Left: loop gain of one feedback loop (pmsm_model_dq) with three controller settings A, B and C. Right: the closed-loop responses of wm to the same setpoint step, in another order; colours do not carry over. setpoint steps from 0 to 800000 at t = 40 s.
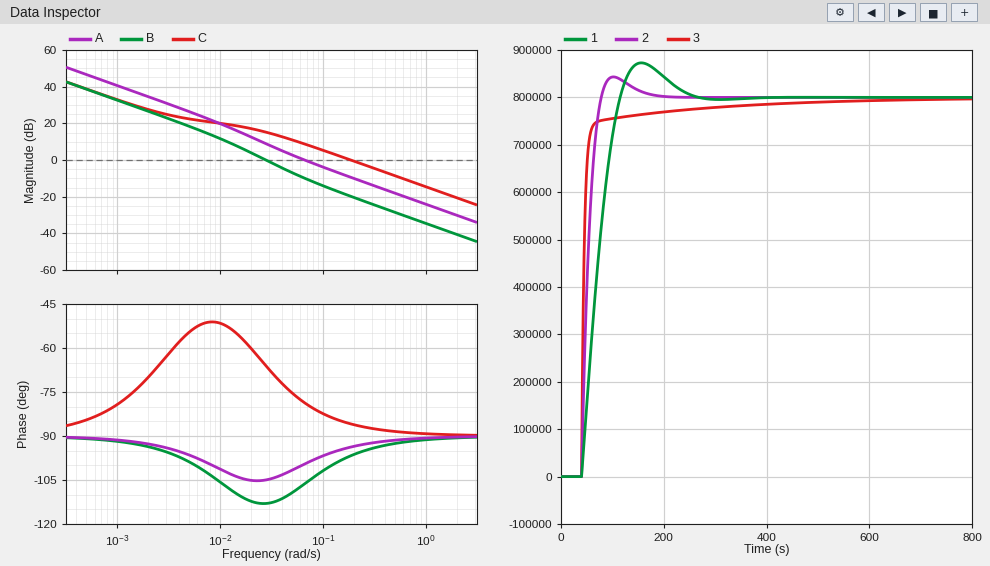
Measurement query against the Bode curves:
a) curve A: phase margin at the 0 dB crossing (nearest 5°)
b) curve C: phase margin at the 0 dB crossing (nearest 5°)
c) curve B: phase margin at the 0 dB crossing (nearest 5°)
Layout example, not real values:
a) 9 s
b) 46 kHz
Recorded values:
a) 80°
b) 95°
c) 65°
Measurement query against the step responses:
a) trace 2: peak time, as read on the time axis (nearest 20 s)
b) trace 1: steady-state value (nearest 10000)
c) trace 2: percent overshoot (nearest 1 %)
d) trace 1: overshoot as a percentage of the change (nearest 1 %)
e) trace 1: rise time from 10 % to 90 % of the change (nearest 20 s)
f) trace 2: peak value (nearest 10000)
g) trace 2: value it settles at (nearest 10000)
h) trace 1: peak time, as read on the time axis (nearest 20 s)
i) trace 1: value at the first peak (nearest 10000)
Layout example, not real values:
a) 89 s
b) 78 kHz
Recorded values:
a) 100 s
b) 800000
c) 5 %
d) 9 %
e) 60 s
f) 840000
g) 800000
h) 160 s
i) 870000
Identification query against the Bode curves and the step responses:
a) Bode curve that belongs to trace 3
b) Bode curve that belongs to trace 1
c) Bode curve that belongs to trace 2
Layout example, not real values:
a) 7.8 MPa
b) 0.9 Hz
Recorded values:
a) C
b) B
c) A
